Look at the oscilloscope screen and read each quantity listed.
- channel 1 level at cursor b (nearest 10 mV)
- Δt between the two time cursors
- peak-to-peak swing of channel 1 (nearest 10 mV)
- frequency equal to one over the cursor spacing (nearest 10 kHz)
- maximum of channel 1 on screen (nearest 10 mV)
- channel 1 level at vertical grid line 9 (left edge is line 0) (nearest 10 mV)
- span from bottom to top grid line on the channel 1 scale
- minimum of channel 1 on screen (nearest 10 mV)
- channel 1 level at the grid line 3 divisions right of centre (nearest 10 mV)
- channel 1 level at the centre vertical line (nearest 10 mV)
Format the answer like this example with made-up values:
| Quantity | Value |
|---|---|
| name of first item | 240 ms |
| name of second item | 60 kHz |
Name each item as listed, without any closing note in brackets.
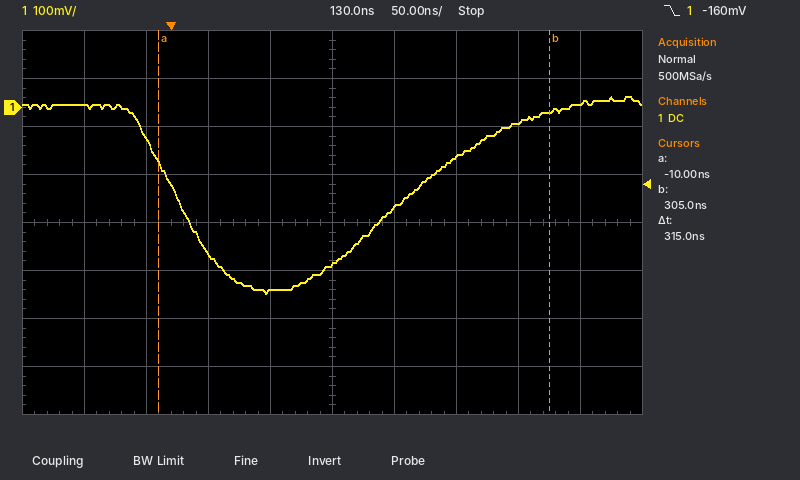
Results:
| Quantity | Value |
|---|---|
| channel 1 level at cursor b | -10 mV |
| Δt between the two time cursors | 315 ns |
| peak-to-peak swing of channel 1 | 410 mV |
| frequency equal to one over the cursor spacing | 3.17 MHz |
| maximum of channel 1 on screen | 20 mV |
| channel 1 level at vertical grid line 9 (left edge is line 0) | 10 mV |
| span from bottom to top grid line on the channel 1 scale | 800 mV |
| minimum of channel 1 on screen | -390 mV |
| channel 1 level at the grid line 3 divisions right of centre | -30 mV |
| channel 1 level at the centre vertical line | -330 mV |
